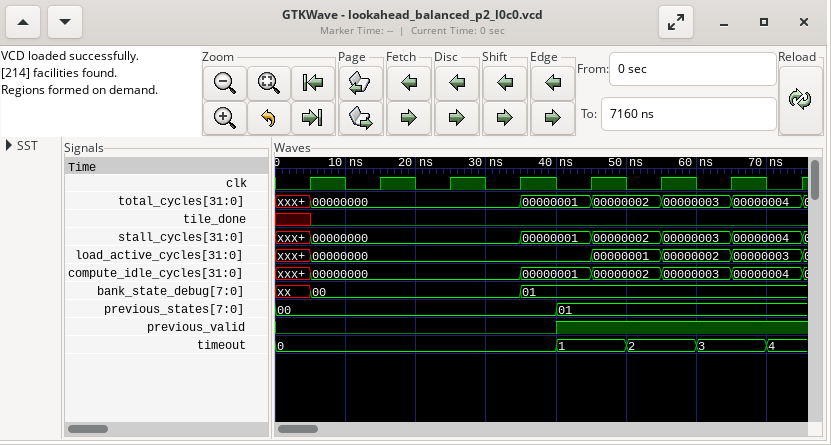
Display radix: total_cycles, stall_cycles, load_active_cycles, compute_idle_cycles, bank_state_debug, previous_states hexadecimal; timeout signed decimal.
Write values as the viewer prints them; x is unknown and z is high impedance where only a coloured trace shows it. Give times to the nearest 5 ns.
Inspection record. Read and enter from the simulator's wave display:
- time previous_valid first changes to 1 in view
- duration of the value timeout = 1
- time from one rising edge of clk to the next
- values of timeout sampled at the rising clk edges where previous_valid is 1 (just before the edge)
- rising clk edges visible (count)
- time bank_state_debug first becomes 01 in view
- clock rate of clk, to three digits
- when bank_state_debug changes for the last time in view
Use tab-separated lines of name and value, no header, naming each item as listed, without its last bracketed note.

time previous_valid first changes to 1 in view	40 ns
duration of the value timeout = 1	10 ns
time from one rising edge of clk to the next	10 ns
values of timeout sampled at the rising clk edges where previous_valid is 1	1, 2, 3, 4
rising clk edges visible	8
time bank_state_debug first becomes 01 in view	35 ns
clock rate of clk, to three digits	100 MHz
when bank_state_debug changes for the last time in view	35 ns
